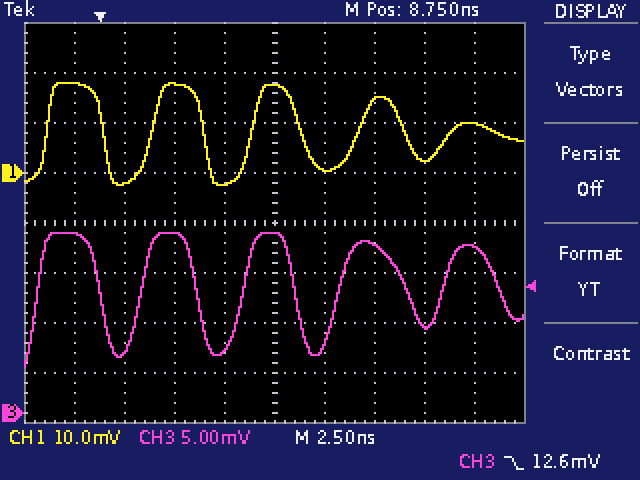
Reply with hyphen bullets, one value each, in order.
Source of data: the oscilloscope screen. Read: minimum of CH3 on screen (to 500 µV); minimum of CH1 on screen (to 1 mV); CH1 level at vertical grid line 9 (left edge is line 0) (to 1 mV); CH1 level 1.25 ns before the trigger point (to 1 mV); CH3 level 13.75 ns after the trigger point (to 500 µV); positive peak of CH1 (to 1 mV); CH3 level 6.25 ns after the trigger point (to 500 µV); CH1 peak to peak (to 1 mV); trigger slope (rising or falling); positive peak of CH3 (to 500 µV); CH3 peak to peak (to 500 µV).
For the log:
- 4.5 mV
- -2 mV
- 10 mV
- 18 mV
- 17.0 mV
- 18 mV
- 6.5 mV
- 20 mV
- falling
- 18.0 mV
- 13.5 mV
